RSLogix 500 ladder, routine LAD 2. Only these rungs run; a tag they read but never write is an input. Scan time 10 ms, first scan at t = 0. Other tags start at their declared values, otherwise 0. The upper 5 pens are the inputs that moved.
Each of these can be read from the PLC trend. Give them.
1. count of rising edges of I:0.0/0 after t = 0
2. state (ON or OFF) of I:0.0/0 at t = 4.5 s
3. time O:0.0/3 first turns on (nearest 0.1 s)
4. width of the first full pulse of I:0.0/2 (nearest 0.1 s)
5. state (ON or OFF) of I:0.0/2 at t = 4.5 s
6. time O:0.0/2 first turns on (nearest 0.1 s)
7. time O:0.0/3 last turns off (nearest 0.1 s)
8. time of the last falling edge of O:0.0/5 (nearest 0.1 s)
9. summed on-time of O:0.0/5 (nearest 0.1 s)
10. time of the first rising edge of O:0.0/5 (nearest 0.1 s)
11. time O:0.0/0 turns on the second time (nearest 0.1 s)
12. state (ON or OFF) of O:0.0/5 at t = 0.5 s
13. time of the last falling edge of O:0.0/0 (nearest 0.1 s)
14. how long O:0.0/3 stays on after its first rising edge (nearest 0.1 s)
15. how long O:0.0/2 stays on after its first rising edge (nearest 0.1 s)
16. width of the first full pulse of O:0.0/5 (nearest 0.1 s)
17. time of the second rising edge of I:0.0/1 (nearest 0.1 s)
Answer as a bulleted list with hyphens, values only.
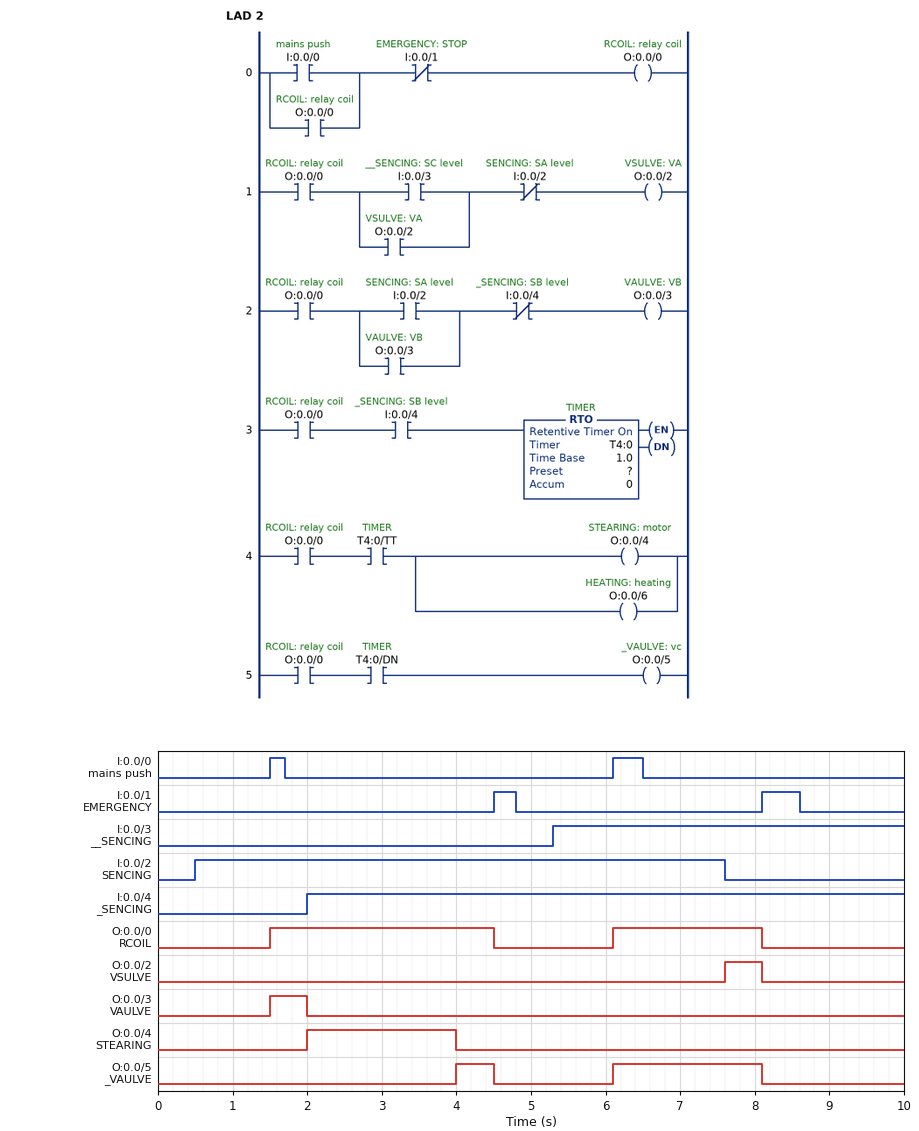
- 2
- OFF
- 1.5 s
- 7.1 s
- ON
- 7.6 s
- 2.0 s
- 8.1 s
- 2.5 s
- 4.0 s
- 6.1 s
- OFF
- 8.1 s
- 0.5 s
- 0.5 s
- 0.5 s
- 8.1 s
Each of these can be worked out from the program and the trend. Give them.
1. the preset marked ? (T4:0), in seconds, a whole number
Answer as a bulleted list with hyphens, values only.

- 2 s
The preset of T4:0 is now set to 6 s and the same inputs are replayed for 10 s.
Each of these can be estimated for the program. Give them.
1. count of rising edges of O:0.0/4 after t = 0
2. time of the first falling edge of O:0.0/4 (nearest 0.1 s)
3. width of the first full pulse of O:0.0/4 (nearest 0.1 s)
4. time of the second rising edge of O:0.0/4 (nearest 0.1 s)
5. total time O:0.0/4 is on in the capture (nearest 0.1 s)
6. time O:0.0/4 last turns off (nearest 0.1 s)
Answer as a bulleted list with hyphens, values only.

- 2
- 4.5 s
- 2.5 s
- 6.1 s
- 4.5 s
- 8.1 s
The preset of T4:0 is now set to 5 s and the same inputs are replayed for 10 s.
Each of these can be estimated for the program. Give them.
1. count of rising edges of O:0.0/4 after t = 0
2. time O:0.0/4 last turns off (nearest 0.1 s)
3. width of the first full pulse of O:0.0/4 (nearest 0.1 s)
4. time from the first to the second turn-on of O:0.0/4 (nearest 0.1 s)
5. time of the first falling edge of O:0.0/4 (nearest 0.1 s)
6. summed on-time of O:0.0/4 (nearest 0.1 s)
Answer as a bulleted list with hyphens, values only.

- 2
- 8.1 s
- 2.5 s
- 4.1 s
- 4.5 s
- 4.5 s
